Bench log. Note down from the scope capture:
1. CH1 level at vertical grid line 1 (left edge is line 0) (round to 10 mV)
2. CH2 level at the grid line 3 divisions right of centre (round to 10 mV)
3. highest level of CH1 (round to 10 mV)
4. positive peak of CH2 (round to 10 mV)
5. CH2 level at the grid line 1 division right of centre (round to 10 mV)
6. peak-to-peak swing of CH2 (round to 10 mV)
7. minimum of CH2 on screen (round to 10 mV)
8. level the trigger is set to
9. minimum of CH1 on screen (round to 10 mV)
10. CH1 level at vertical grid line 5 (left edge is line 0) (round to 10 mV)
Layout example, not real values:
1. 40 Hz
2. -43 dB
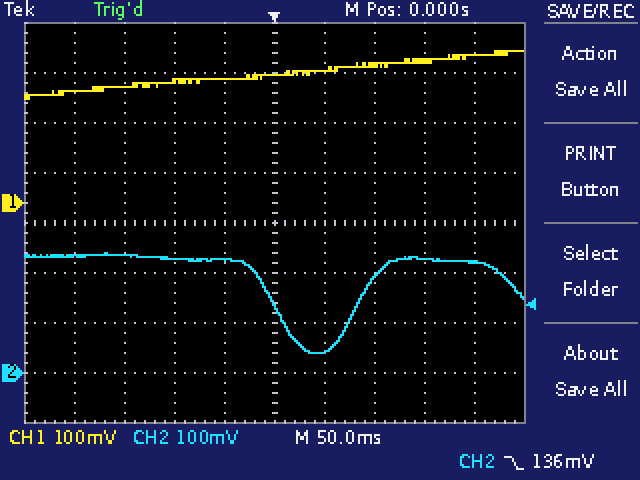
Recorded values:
1. 220 mV
2. 230 mV
3. 300 mV
4. 240 mV
5. 40 mV
6. 200 mV
7. 40 mV
8. 136 mV
9. 210 mV
10. 260 mV
